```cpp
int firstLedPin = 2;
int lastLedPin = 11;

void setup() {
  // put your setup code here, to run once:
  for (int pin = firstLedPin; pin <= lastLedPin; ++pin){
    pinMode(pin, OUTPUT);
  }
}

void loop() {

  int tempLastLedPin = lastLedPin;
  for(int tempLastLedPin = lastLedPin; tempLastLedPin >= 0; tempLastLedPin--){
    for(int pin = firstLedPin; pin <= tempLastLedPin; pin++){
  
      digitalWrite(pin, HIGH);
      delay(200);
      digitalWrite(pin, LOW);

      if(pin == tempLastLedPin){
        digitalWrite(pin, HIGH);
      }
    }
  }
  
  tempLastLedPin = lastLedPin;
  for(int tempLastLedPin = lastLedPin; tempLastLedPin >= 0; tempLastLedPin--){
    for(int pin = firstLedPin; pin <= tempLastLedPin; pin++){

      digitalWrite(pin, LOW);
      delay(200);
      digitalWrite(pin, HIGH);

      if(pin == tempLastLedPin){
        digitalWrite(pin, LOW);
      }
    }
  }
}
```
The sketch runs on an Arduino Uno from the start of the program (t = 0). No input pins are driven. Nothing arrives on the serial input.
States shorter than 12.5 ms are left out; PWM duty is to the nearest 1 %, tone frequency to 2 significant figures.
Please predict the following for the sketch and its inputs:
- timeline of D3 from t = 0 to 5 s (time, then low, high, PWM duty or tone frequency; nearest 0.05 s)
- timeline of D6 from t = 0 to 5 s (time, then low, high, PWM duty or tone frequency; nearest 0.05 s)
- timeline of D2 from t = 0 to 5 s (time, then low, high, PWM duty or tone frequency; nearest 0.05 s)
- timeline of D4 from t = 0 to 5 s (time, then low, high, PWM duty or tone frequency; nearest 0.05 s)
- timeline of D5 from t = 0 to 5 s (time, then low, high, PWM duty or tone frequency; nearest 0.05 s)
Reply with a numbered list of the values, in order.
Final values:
1. 0 s low; 0.2 s high; 0.4 s low; 2.2 s high; 2.4 s low; 4 s high; 4.2 s low
2. 0 s low; 0.8 s high; 1 s low; 2.8 s high; 3 s low; 4.6 s high; 4.8 s low
3. 0 s high; 0.2 s low; 2 s high; 2.2 s low; 3.8 s high; 4 s low
4. 0 s low; 0.4 s high; 0.6 s low; 2.4 s high; 2.6 s low; 4.2 s high; 4.4 s low
5. 0 s low; 0.6 s high; 0.8 s low; 2.6 s high; 2.8 s low; 4.4 s high; 4.6 s low
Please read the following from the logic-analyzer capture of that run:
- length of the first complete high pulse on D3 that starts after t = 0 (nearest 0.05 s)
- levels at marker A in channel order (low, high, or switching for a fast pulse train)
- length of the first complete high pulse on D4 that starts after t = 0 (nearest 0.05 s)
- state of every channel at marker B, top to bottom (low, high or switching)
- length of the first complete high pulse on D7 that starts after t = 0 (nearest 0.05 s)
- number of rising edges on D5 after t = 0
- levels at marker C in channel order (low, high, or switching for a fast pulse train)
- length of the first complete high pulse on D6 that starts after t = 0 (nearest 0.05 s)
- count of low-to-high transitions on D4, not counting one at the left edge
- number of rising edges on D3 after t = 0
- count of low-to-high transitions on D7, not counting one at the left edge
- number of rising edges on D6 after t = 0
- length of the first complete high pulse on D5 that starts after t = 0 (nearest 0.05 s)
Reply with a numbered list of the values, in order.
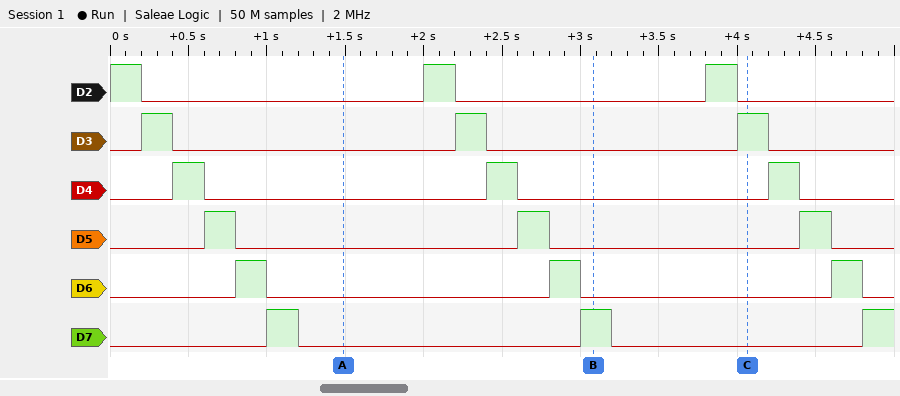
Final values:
1. 0.20 s
2. D2 low, D3 low, D4 low, D5 low, D6 low, D7 low
3. 0.20 s
4. D2 low, D3 low, D4 low, D5 low, D6 low, D7 high
5. 0.20 s
6. 3
7. D2 low, D3 high, D4 low, D5 low, D6 low, D7 low
8. 0.20 s
9. 3
10. 3
11. 3
12. 3
13. 0.20 s
